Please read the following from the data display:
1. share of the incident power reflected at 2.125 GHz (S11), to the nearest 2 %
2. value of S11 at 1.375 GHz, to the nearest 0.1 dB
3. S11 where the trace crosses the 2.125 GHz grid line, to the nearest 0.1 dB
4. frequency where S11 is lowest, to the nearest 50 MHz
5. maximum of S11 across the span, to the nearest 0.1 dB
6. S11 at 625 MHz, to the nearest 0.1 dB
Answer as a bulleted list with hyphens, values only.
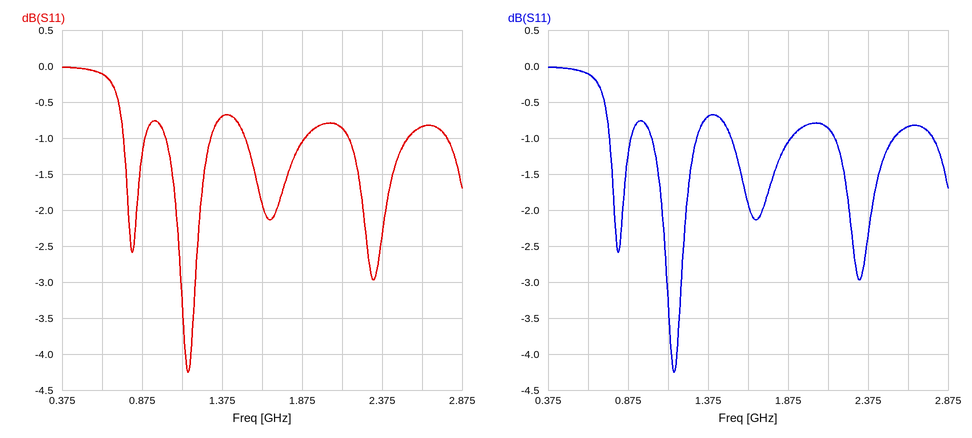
- 82 %
- -0.7 dB
- -0.9 dB
- 1.15 GHz
- 0.0 dB
- -0.1 dB
